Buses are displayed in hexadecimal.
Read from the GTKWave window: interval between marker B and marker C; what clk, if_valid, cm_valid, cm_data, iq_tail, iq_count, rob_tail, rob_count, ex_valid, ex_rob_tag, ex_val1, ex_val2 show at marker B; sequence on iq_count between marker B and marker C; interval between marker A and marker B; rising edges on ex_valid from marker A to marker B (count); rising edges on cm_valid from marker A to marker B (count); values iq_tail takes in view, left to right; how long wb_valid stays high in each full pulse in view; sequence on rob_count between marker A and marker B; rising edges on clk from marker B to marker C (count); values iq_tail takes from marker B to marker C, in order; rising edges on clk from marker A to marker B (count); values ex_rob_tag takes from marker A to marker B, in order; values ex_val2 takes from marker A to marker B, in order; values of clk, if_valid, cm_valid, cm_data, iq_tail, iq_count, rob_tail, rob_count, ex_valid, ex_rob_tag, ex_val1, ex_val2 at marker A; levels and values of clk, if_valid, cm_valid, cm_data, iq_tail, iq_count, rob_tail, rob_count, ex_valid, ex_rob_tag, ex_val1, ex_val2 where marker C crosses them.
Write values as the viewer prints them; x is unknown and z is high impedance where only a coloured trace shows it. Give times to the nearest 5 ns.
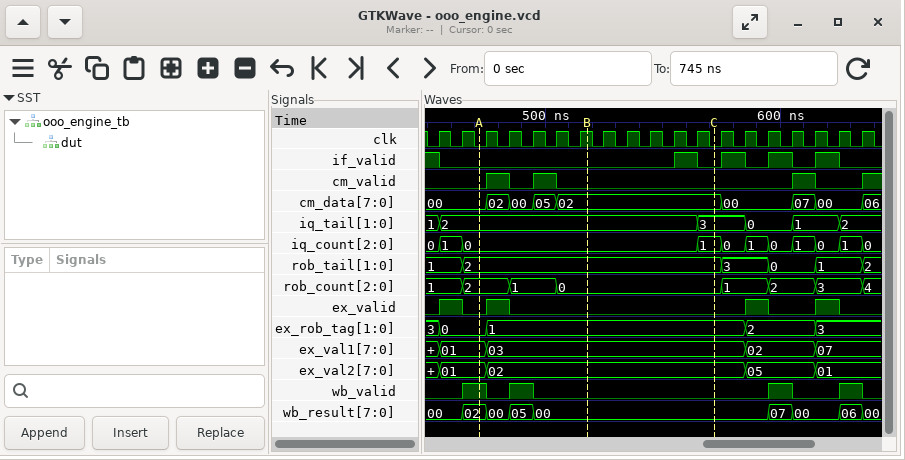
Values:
55 ns
clk=1, if_valid=0, cm_valid=0, cm_data=02, iq_tail=2, iq_count=0, rob_tail=2, rob_count=0, ex_valid=0, ex_rob_tag=1, ex_val1=03, ex_val2=02
0, 1
45 ns
1
2
1, 2, 3, 0, 1, 2
10 ns, 10 ns, 10 ns, 10 ns
2, 1, 0
5
2, 3
5
0, 1
01, 02
clk=0, if_valid=0, cm_valid=0, cm_data=00, iq_tail=2, iq_count=0, rob_tail=2, rob_count=2, ex_valid=0, ex_rob_tag=0, ex_val1=01, ex_val2=01
clk=0, if_valid=0, cm_valid=0, cm_data=02, iq_tail=3, iq_count=1, rob_tail=2, rob_count=0, ex_valid=0, ex_rob_tag=1, ex_val1=03, ex_val2=02
